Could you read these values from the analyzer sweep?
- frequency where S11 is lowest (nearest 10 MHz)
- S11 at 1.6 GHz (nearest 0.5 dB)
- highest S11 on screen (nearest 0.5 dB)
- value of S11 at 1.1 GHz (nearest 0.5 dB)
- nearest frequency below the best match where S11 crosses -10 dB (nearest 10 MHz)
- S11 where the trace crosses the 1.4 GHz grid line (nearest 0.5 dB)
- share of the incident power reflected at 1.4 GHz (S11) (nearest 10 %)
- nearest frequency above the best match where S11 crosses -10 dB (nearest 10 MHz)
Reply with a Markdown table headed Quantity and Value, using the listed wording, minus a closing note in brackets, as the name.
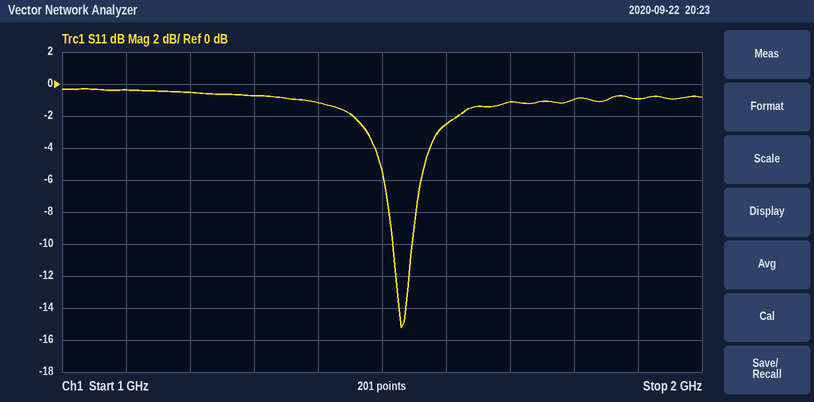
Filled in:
| Quantity | Value |
|---|---|
| frequency where S11 is lowest | 1.53 GHz |
| S11 at 1.6 GHz | -2.5 dB |
| highest S11 on screen | -0.5 dB |
| value of S11 at 1.1 GHz | -0.5 dB |
| nearest frequency below the best match where S11 crosses -10 dB | 1.52 GHz |
| S11 where the trace crosses the 1.4 GHz grid line | -1.0 dB |
| share of the incident power reflected at 1.4 GHz (S11) | 80 % |
| nearest frequency above the best match where S11 crosses -10 dB | 1.55 GHz |
